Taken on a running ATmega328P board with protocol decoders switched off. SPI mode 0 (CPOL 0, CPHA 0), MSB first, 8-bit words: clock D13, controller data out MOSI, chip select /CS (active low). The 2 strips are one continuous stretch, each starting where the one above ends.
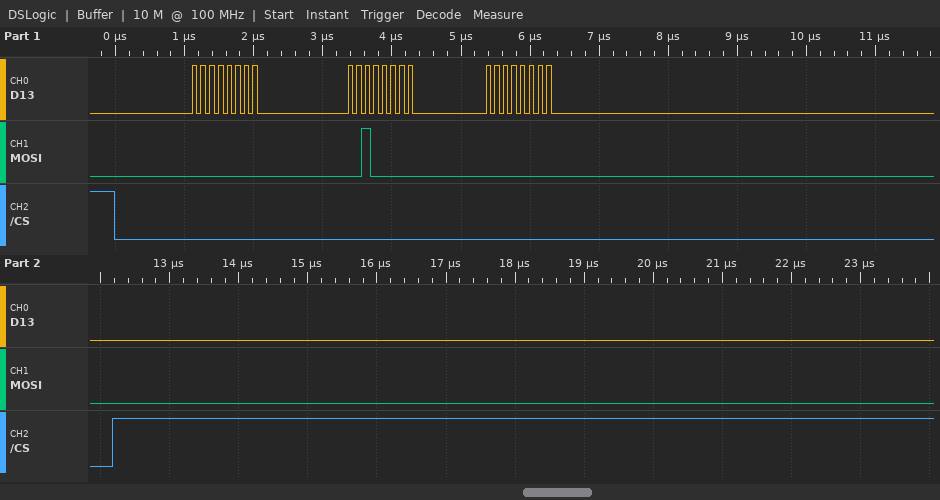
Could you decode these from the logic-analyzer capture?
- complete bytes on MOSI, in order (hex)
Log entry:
00 20 00
